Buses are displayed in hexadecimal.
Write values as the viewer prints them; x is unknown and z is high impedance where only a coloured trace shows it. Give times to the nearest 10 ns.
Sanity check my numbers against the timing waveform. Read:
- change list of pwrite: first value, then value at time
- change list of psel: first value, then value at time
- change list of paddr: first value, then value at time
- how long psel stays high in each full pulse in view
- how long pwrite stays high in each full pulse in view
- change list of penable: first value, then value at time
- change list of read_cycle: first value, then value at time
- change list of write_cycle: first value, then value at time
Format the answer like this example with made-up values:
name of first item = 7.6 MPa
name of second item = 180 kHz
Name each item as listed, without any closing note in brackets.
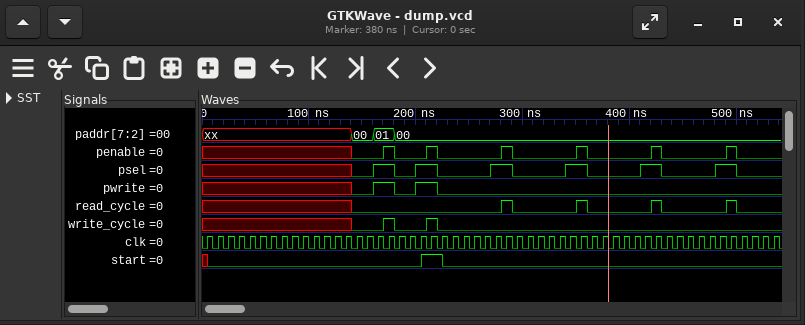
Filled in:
change list of pwrite: first value, then value at time = x, 0 at 140 ns, 1 at 160 ns, 0 at 180 ns, 1 at 200 ns, 0 at 220 ns
change list of psel: first value, then value at time = x, 0 at 140 ns, 1 at 160 ns, 0 at 180 ns, 1 at 200 ns, 0 at 220 ns, 1 at 270 ns, 0 at 290 ns, 1 at 340 ns, 0 at 360 ns, 1 at 410 ns, 0 at 430 ns, 1 at 480 ns, 0 at 500 ns
change list of paddr: first value, then value at time = xx, 00 at 140 ns, 01 at 160 ns, 00 at 180 ns
how long psel stays high in each full pulse in view = 20 ns, 20 ns, 20 ns, 20 ns, 20 ns, 20 ns
how long pwrite stays high in each full pulse in view = 20 ns, 20 ns
change list of penable: first value, then value at time = x, 0 at 140 ns, 1 at 170 ns, 0 at 180 ns, 1 at 210 ns, 0 at 220 ns, 1 at 280 ns, 0 at 290 ns, 1 at 350 ns, 0 at 360 ns, 1 at 420 ns, 0 at 430 ns, 1 at 490 ns, 0 at 500 ns
change list of read_cycle: first value, then value at time = x, 0 at 140 ns, 1 at 280 ns, 0 at 290 ns, 1 at 350 ns, 0 at 360 ns, 1 at 420 ns, 0 at 430 ns, 1 at 490 ns, 0 at 500 ns
change list of write_cycle: first value, then value at time = x, 0 at 140 ns, 1 at 170 ns, 0 at 180 ns, 1 at 210 ns, 0 at 220 ns
